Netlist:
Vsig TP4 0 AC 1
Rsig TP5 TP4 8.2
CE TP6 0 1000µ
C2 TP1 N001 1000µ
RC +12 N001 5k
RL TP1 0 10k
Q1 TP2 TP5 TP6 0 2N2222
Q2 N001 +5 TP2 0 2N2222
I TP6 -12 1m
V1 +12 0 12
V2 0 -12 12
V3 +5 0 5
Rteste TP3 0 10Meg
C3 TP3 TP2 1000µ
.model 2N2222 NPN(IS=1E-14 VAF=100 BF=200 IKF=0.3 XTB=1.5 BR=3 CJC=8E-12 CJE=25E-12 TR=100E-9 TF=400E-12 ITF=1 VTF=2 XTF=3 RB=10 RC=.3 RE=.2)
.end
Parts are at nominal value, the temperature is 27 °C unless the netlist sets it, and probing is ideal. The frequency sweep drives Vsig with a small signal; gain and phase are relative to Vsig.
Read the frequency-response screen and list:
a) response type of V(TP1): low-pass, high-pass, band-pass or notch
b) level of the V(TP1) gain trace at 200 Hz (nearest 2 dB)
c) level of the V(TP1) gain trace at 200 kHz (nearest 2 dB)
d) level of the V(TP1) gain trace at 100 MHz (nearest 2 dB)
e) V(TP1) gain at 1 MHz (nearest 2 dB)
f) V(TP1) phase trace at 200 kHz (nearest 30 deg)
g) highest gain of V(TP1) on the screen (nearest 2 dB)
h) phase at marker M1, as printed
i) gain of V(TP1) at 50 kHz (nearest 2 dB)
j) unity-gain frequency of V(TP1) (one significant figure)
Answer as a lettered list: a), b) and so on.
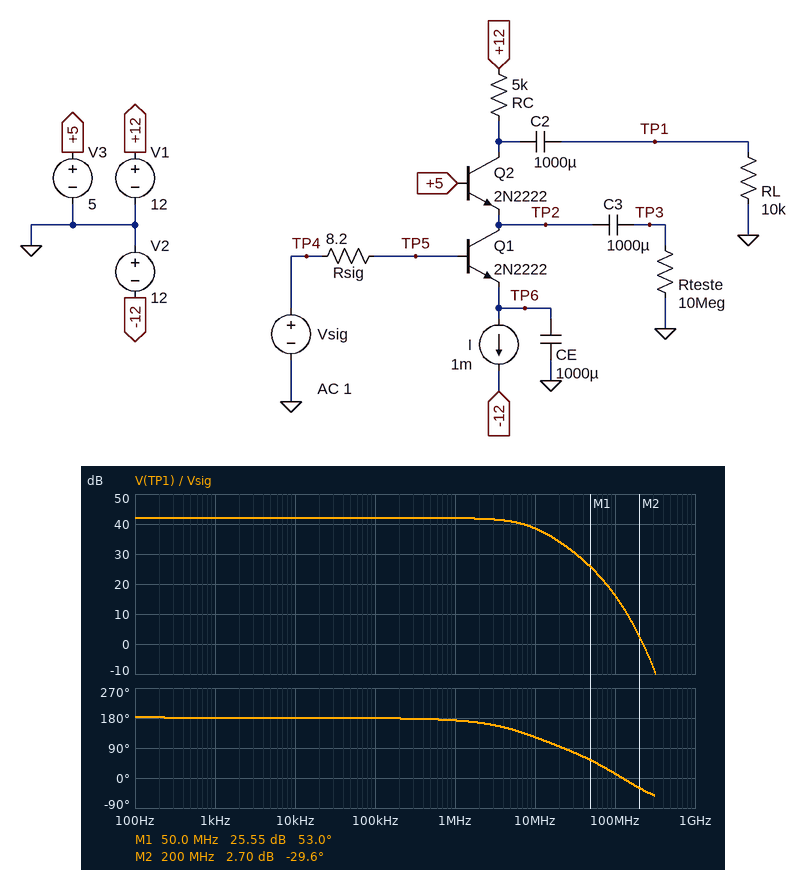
a) low-pass
b) 42 dB
c) 42 dB
d) 16 dB
e) 42 dB
f) 180 deg
g) 42 dB
h) 53.0 deg
i) 42 dB
j) 200 MHz
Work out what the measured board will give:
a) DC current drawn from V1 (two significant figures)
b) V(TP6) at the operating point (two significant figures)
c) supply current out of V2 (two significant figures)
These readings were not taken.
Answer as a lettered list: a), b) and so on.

a) 990 µA
b) -650 mV
c) 1.0 mA
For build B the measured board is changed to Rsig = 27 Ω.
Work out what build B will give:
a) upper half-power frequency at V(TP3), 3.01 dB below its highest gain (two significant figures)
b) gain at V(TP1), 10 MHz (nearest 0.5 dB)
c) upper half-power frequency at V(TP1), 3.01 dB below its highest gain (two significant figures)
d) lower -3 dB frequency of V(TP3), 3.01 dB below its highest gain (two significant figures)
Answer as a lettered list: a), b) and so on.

a) 60 MHz
b) 38.5 dB
c) 9.0 MHz
d) 10 Hz
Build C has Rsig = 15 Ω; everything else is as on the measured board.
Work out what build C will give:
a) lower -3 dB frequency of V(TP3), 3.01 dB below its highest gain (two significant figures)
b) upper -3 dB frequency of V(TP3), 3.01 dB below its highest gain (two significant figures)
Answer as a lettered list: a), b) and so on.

a) 11 Hz
b) 74 MHz
